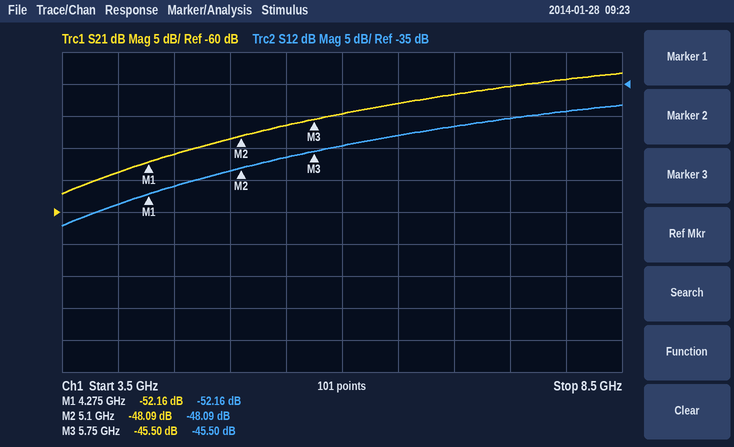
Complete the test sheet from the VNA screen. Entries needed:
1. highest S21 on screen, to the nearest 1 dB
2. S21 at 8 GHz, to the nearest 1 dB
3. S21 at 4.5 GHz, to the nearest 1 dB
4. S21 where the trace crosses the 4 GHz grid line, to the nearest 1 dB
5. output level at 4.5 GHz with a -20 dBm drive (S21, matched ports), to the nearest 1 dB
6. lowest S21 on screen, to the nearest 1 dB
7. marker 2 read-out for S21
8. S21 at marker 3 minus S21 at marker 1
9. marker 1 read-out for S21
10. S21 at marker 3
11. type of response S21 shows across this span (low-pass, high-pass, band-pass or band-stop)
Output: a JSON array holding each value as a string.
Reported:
["-38 dB", "-39 dB", "-51 dB", "-54 dB", "-71 dBm", "-57 dB", "-48.09 dB", "6.66 dB", "-52.16 dB", "-45.50 dB", "high-pass"]
